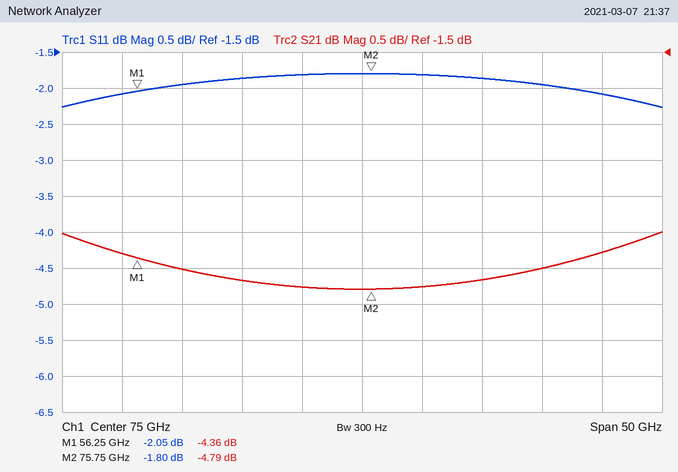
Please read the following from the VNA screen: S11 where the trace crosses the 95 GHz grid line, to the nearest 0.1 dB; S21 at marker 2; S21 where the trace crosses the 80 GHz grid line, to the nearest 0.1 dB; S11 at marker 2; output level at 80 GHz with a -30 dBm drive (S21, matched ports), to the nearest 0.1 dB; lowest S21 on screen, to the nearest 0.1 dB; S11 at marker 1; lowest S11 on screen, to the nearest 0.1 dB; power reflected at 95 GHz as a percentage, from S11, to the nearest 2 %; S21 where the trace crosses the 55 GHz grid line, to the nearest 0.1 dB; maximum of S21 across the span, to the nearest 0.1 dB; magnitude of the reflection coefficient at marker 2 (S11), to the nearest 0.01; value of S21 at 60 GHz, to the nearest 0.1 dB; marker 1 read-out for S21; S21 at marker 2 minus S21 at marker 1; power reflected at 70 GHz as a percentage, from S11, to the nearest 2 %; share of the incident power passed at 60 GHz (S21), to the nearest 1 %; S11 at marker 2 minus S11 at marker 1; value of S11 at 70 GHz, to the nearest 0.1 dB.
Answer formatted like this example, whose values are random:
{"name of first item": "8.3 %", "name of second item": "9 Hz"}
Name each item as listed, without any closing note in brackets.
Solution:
{"S11 where the trace crosses the 95 GHz grid line, to the nearest 0.1 dB": "-2.1 dB", "S21 at marker 2": "-4.79 dB", "S21 where the trace crosses the 80 GHz grid line, to the nearest 0.1 dB": "-4.8 dB", "S11 at marker 2": "-1.80 dB", "output level at 80 GHz with a -30 dBm drive (S21, matched ports), to the nearest 0.1 dB": "-34.8 dBm", "lowest S21 on screen, to the nearest 0.1 dB": "-4.8 dB", "S11 at marker 1": "-2.05 dB", "lowest S11 on screen, to the nearest 0.1 dB": "-2.3 dB", "power reflected at 95 GHz as a percentage, from S11, to the nearest 2 %": "62 %", "S21 where the trace crosses the 55 GHz grid line, to the nearest 0.1 dB": "-4.3 dB", "maximum of S21 across the span, to the nearest 0.1 dB": "-4.0 dB", "magnitude of the reflection coefficient at marker 2 (S11), to the nearest 0.01": "0.81", "value of S21 at 60 GHz, to the nearest 0.1 dB": "-4.5 dB", "marker 1 read-out for S21": "-4.36 dB", "S21 at marker 2 minus S21 at marker 1": "-0.43 dB", "power reflected at 70 GHz as a percentage, from S11, to the nearest 2 %": "66 %", "share of the incident power passed at 60 GHz (S21), to the nearest 1 %": "35 %", "S11 at marker 2 minus S11 at marker 1": "0.25 dB", "value of S11 at 70 GHz, to the nearest 0.1 dB": "-1.8 dB"}
